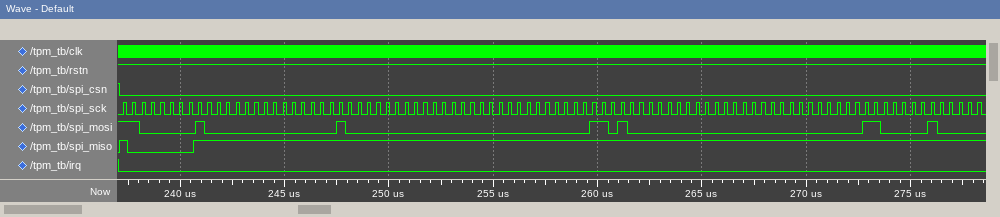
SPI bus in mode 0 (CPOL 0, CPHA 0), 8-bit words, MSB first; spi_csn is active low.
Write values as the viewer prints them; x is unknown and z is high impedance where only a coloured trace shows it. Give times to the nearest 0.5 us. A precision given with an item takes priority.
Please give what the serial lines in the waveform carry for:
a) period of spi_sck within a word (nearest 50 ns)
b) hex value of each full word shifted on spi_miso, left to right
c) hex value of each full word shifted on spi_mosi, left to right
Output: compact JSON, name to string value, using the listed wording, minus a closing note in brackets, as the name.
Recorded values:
{"period of spi_sck within a word": "450 ns", "hex value of each full word shifted on spi_miso, left to right": "80, FF, FF, FF, FF, FF, FF, FF, FF, FF, FF", "hex value of each full word shifted on spi_mosi, left to right": "C0, 80, 01, 00, 00, 00, 34, 00, 00, 01, 82"}
